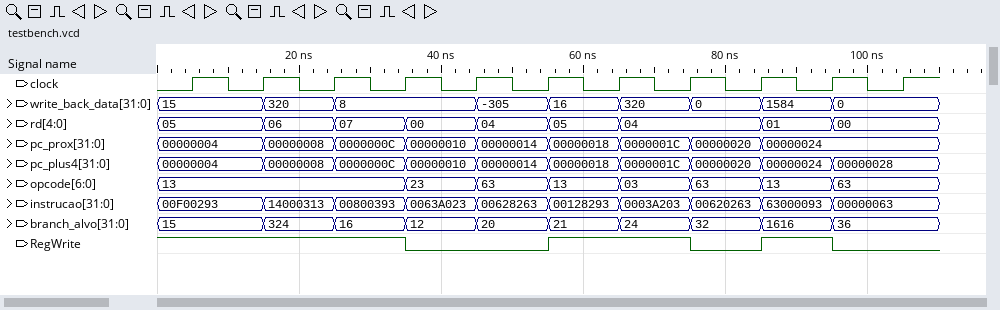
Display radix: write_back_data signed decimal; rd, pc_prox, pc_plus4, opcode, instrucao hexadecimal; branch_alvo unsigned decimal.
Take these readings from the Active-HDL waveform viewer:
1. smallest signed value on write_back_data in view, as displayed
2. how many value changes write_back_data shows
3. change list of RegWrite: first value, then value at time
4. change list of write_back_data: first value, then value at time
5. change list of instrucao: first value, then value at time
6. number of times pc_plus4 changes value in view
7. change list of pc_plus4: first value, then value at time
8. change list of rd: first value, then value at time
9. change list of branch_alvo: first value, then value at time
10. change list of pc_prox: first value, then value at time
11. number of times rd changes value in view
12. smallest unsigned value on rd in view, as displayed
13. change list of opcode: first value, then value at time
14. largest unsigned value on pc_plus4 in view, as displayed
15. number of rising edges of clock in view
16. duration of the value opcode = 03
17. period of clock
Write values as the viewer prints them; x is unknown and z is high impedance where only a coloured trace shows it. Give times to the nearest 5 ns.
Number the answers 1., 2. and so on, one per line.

1. -305
2. 8
3. 1, 0 at 35 ns, 1 at 55 ns, 0 at 75 ns, 1 at 85 ns, 0 at 95 ns
4. 15, 320 at 15 ns, 8 at 25 ns, -305 at 45 ns, 16 at 55 ns, 320 at 65 ns, 0 at 75 ns, 1584 at 85 ns, 0 at 95 ns
5. 00F00293, 14000313 at 15 ns, 00800393 at 25 ns, 0063A023 at 35 ns, 00628263 at 45 ns, 00128293 at 55 ns, 0003A203 at 65 ns, 00620263 at 75 ns, 63000093 at 85 ns, 00000063 at 95 ns
6. 9
7. 00000004, 00000008 at 15 ns, 0000000C at 25 ns, 00000010 at 35 ns, 00000014 at 45 ns, 00000018 at 55 ns, 0000001C at 65 ns, 00000020 at 75 ns, 00000024 at 85 ns, 00000028 at 95 ns
8. 05, 06 at 15 ns, 07 at 25 ns, 00 at 35 ns, 04 at 45 ns, 05 at 55 ns, 04 at 65 ns, 01 at 85 ns, 00 at 95 ns
9. 15, 324 at 15 ns, 16 at 25 ns, 12 at 35 ns, 20 at 45 ns, 21 at 55 ns, 24 at 65 ns, 32 at 75 ns, 1616 at 85 ns, 36 at 95 ns
10. 00000004, 00000008 at 15 ns, 0000000C at 25 ns, 00000010 at 35 ns, 00000014 at 45 ns, 00000018 at 55 ns, 0000001C at 65 ns, 00000020 at 75 ns, 00000024 at 85 ns
11. 8
12. 00
13. 13, 23 at 35 ns, 63 at 45 ns, 13 at 55 ns, 03 at 65 ns, 63 at 75 ns, 13 at 85 ns, 63 at 95 ns
14. 00000028
15. 11
16. 10 ns
17. 10 ns
